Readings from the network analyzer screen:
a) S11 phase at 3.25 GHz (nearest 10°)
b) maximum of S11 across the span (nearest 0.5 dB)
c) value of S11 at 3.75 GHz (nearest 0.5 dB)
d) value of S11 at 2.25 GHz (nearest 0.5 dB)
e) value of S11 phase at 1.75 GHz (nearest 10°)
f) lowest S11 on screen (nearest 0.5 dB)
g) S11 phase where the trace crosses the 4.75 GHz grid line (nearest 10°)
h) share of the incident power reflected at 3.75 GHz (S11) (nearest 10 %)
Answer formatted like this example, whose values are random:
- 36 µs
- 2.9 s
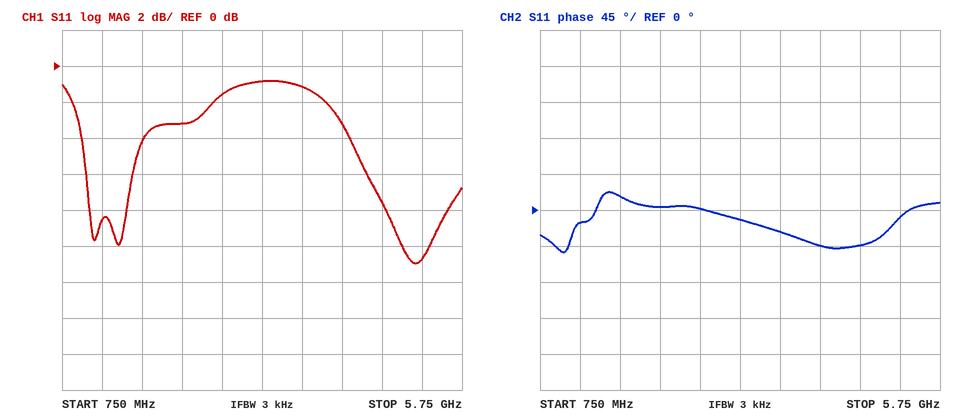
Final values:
- -10°
- -1.0 dB
- -1.0 dB
- -3.0 dB
- 20°
- -11.0 dB
- -40°
- 80 %
